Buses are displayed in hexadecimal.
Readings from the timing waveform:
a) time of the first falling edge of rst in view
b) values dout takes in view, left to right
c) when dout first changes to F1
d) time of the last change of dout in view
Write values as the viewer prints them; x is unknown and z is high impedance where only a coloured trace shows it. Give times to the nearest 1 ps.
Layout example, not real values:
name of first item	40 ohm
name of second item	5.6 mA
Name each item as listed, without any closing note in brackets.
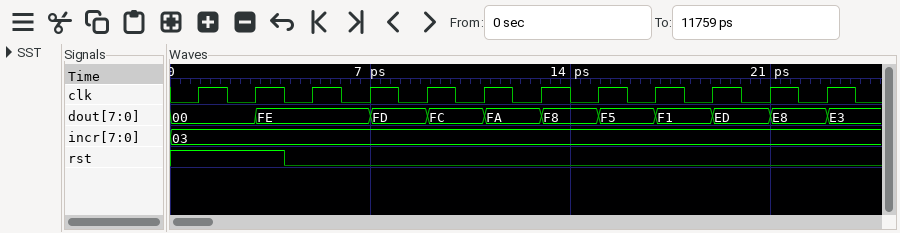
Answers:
time of the first falling edge of rst in view	4 ps
values dout takes in view, left to right	00, FE, FD, FC, FA, F8, F5, F1, ED, E8, E3
when dout first changes to F1	17 ps
time of the last change of dout in view	23 ps
